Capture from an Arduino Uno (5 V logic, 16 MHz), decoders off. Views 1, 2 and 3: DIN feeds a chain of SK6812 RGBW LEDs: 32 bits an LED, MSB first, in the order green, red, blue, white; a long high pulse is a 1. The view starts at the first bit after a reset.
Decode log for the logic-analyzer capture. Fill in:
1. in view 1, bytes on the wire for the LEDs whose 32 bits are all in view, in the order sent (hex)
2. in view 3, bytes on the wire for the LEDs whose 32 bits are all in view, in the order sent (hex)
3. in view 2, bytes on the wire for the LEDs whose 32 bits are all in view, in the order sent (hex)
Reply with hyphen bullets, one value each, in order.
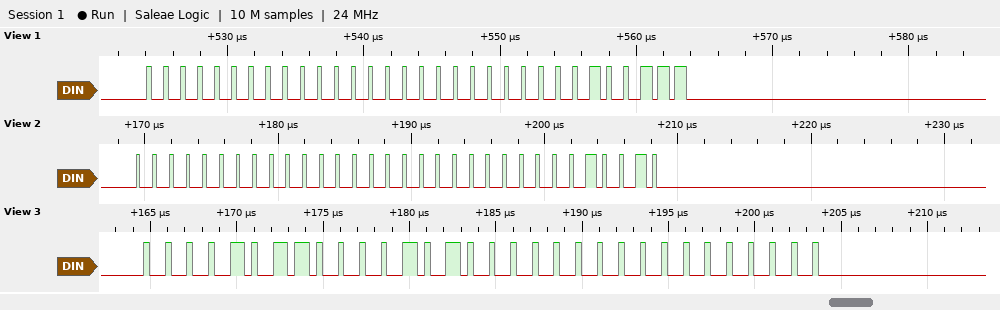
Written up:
- 00 00 00 27
- 0B 0A 00 00
- 00 00 00 12
